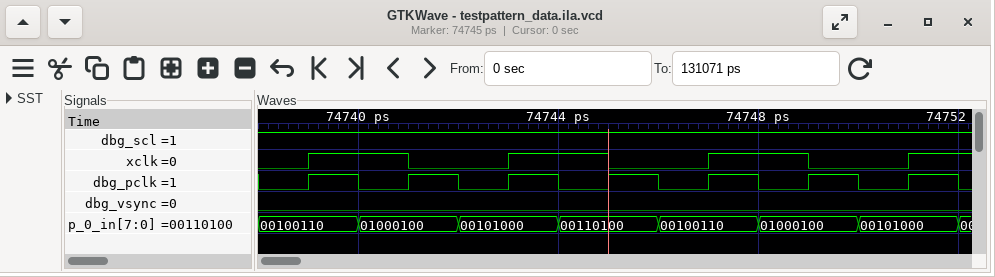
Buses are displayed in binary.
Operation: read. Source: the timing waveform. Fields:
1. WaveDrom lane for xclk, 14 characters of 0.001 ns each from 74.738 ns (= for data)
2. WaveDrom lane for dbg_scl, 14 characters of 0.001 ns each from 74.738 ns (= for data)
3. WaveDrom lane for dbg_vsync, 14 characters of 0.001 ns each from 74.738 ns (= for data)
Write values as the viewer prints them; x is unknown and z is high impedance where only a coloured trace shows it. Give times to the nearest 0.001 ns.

{name: 'xclk', wave: '01.0.1.0.1.0.1'}
{name: 'dbg_scl', wave: '1.............'}
{name: 'dbg_vsync', wave: '0.............'}
